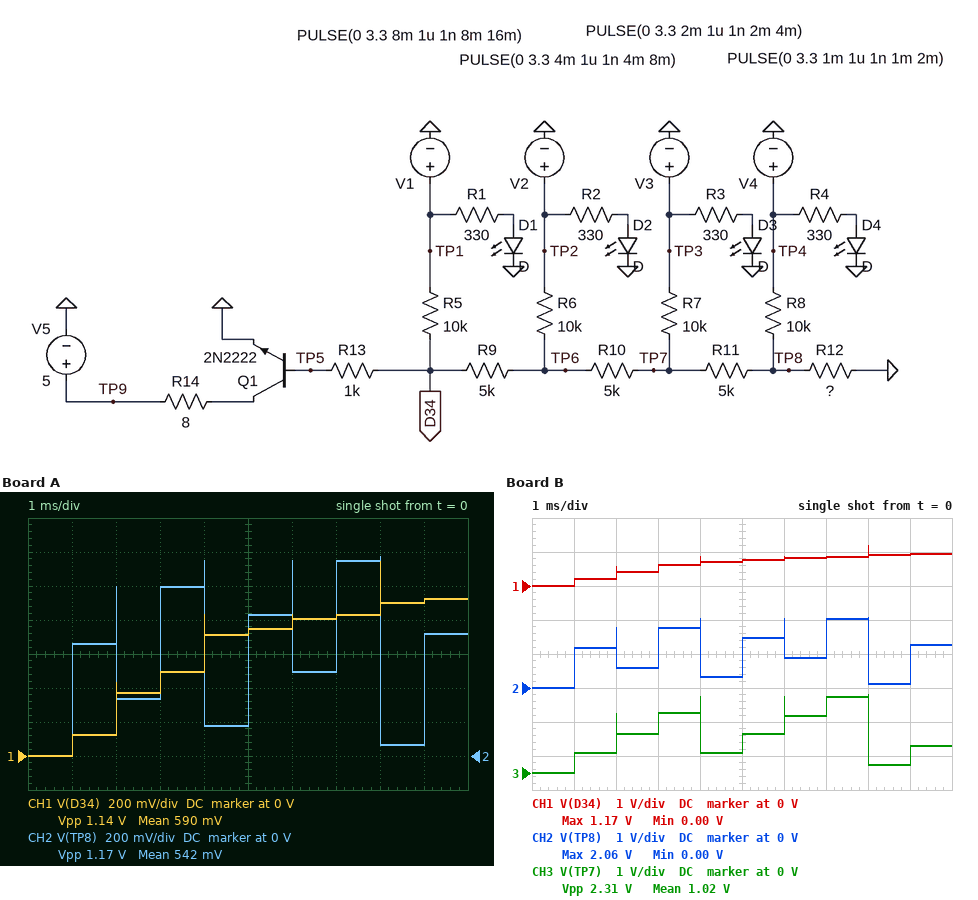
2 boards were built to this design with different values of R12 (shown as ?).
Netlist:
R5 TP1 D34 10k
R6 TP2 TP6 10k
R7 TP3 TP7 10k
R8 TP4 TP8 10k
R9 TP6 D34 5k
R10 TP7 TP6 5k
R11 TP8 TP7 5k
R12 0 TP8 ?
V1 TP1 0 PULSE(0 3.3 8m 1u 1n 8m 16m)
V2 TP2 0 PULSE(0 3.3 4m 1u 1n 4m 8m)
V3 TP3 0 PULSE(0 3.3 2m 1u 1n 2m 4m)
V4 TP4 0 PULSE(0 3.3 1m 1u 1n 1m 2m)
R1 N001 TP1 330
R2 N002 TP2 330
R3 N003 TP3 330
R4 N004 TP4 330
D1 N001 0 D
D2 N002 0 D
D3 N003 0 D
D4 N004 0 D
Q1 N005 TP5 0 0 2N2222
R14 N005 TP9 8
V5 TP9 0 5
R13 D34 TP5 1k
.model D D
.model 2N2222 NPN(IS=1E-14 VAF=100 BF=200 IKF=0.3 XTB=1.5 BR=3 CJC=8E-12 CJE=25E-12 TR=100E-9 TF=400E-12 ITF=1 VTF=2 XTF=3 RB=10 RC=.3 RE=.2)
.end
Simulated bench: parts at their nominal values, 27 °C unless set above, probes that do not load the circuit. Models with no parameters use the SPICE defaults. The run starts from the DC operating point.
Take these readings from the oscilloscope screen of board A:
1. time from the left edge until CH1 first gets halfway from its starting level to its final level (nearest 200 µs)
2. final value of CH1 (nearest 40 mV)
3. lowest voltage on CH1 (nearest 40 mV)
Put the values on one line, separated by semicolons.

3.0 ms; 920 mV; 0 V
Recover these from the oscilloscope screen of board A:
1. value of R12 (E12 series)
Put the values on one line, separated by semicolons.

3.3 kΩ
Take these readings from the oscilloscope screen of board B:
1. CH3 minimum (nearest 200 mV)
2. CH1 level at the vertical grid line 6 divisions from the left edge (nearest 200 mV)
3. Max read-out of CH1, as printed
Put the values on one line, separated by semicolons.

0 V; 800 mV; 1.17 V
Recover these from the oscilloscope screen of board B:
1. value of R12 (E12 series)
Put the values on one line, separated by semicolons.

12 kΩ
